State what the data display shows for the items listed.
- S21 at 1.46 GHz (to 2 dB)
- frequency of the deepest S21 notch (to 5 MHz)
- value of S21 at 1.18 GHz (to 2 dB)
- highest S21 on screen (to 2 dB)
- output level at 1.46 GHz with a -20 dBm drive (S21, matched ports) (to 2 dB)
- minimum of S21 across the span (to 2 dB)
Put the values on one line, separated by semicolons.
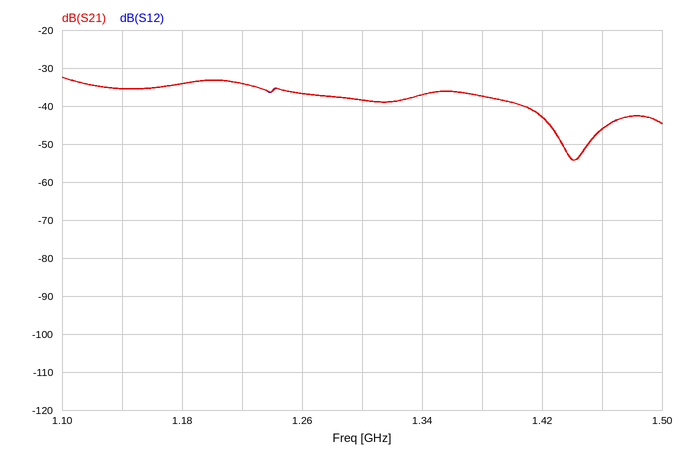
-46 dB; 1.440 GHz; -34 dB; -32 dB; -66 dBm; -54 dB
